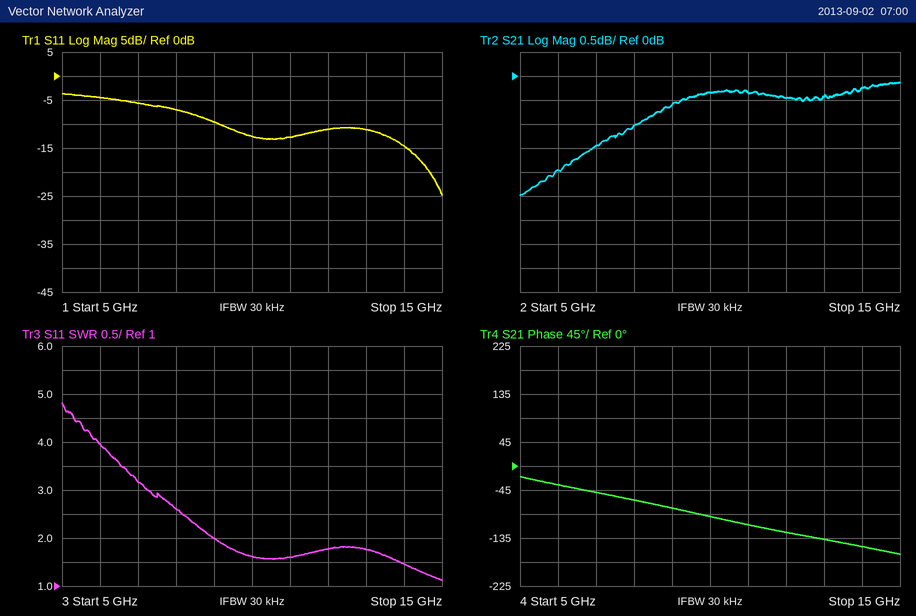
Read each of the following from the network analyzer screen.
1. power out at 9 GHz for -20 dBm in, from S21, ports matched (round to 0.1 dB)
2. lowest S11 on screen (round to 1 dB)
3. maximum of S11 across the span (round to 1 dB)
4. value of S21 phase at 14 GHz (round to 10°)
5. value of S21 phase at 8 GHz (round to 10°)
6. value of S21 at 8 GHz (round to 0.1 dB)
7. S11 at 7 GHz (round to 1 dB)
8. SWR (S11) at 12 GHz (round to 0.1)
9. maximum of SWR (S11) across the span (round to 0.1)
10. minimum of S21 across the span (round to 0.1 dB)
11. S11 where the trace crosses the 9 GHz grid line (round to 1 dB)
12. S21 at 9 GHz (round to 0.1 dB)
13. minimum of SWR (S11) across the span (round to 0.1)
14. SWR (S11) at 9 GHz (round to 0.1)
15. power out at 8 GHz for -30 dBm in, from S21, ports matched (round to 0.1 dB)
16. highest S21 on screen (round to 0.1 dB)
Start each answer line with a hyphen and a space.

- -20.6 dBm
- -25 dB
- -4 dB
- -150°
- -60°
- -1.0 dB
- -6 dB
- 1.8
- 4.8
- -2.5 dB
- -10 dB
- -0.6 dB
- 1.1
- 2.0
- -31.0 dBm
- -0.1 dB
